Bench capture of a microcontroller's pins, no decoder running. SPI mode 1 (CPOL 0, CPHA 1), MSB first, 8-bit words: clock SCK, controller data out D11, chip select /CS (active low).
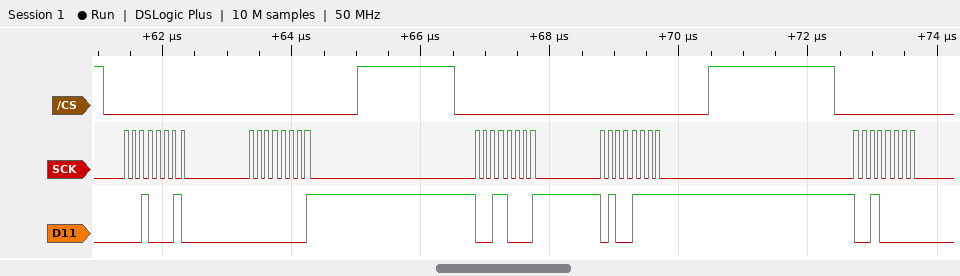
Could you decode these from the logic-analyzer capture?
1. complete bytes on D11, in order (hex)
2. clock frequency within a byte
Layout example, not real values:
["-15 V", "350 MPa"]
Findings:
["22 01 31 4F 20", "8 MHz"]
